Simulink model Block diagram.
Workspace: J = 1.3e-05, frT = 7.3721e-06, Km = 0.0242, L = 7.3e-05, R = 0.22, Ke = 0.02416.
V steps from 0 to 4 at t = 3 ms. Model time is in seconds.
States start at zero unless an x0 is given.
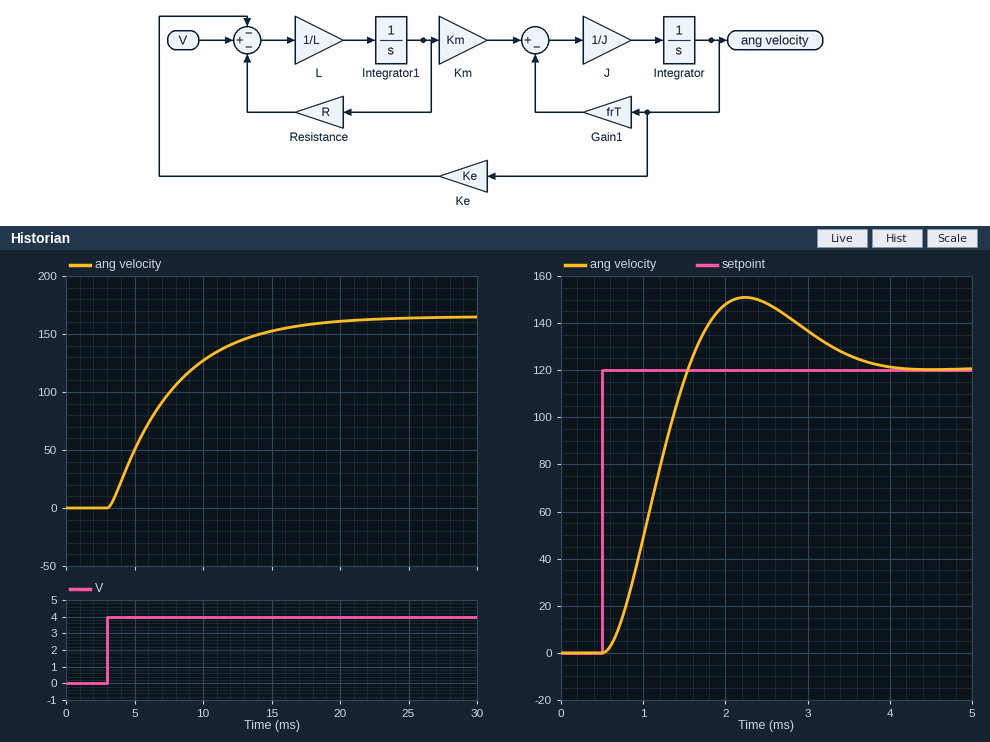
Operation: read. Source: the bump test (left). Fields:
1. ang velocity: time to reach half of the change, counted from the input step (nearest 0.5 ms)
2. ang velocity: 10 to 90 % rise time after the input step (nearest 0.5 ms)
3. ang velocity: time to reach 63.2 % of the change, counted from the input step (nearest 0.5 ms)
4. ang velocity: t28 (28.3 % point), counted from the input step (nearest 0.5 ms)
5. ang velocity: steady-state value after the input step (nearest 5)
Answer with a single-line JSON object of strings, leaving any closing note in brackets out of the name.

{"ang velocity: time to reach half of the change, counted from the input step": "3.5 ms", "ang velocity: 10 to 90 % rise time after the input step": "10.0 ms", "ang velocity: time to reach 63.2 % of the change, counted from the input step": "5.0 ms", "ang velocity: t28 (28.3 % point), counted from the input step": "2.0 ms", "ang velocity: steady-state value after the input step": "165"}
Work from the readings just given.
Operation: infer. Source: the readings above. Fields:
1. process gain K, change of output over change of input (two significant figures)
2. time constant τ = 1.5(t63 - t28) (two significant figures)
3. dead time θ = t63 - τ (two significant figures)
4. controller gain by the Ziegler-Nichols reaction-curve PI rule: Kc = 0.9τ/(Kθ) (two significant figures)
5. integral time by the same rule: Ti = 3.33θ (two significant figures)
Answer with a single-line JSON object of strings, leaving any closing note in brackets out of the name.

{"process gain K, change of output over change of input": "41", "time constant τ = 1.5(t63 - t28)": "4.5 ms", "dead time θ = t63 - τ": "0.50 ms", "controller gain by the Ziegler-Nichols reaction-curve PI rule: Kc = 0.9τ/(Kθ)": "0.20", "integral time by the same rule: Ti = 3.33θ": "1.7 ms"}
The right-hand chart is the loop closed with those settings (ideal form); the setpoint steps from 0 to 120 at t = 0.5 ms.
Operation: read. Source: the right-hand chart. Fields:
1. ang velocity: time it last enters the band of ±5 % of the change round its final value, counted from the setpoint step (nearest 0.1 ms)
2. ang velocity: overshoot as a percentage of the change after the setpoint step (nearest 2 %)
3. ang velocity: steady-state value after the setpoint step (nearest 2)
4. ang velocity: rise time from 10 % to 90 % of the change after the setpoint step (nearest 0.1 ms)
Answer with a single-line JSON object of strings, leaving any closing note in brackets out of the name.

{"ang velocity: time it last enters the band of ±5 % of the change round its final value, counted from the setpoint step": "3.0 ms", "ang velocity: overshoot as a percentage of the change after the setpoint step": "26 %", "ang velocity: steady-state value after the setpoint step": "120", "ang velocity: rise time from 10 % to 90 % of the change after the setpoint step": "0.7 ms"}
